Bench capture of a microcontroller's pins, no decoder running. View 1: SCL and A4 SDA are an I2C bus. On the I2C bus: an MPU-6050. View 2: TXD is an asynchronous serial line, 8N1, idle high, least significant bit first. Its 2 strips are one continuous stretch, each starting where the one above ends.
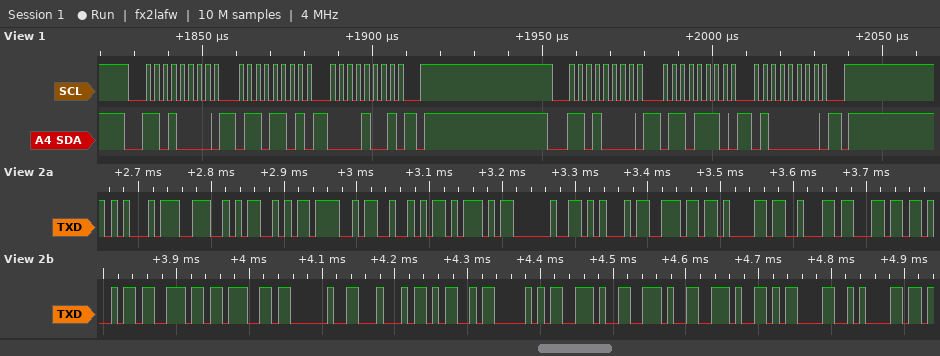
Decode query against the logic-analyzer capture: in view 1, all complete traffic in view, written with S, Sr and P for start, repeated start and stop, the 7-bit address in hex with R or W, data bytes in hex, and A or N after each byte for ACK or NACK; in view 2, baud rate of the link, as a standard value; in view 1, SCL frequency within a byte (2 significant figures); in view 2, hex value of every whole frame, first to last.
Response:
S 68W A 6D A 09 A P S 68W A 6E A 40 A P
115200 baud
400 kHz
45 4E 53 4F 52 5D 20 45 6E 61 62 6C 69 6E 67 20 44 4D 50 2E 2E 2E 0D 0A
